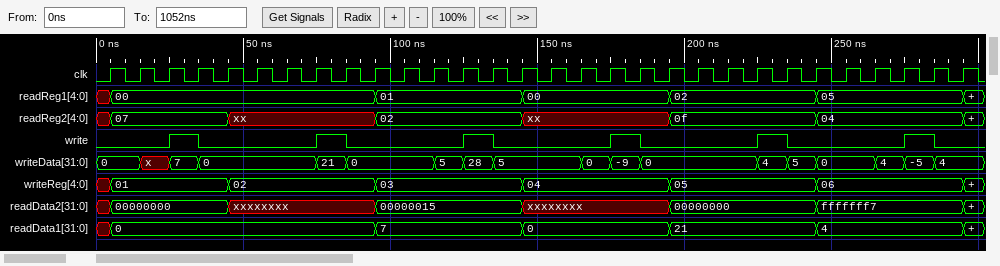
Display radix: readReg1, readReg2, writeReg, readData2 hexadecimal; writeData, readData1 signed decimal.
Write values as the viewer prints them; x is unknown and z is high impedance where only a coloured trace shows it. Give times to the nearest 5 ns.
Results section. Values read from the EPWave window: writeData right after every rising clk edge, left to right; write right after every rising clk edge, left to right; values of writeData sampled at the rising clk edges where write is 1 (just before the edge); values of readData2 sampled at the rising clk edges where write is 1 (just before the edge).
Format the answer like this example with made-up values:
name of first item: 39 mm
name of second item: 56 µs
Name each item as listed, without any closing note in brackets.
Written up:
writeData right after every rising clk edge, left to right: 0, x, 7, 0, 0, 0, 0, 21, 0, 0, 0, 5, 28, 5, 5, 5, 0, -9, 0, 0, 0, 0, 4, 5, 0, 0, 4, -5, 4, 4
write right after every rising clk edge, left to right: 0 0 1 0 0 0 0 1 0 0 0 0 1 0 0 0 0 1 0 0 0 0 1 0 0 0 0 1 0 0
values of writeData sampled at the rising clk edges where write is 1: 7, 21, 28, -9, 4, -5
values of readData2 sampled at the rising clk edges where write is 1: 00000000, xxxxxxxx, 00000015, xxxxxxxx, 00000000, fffffff7
